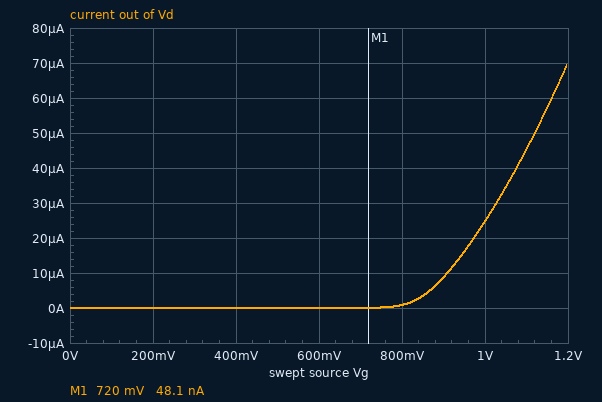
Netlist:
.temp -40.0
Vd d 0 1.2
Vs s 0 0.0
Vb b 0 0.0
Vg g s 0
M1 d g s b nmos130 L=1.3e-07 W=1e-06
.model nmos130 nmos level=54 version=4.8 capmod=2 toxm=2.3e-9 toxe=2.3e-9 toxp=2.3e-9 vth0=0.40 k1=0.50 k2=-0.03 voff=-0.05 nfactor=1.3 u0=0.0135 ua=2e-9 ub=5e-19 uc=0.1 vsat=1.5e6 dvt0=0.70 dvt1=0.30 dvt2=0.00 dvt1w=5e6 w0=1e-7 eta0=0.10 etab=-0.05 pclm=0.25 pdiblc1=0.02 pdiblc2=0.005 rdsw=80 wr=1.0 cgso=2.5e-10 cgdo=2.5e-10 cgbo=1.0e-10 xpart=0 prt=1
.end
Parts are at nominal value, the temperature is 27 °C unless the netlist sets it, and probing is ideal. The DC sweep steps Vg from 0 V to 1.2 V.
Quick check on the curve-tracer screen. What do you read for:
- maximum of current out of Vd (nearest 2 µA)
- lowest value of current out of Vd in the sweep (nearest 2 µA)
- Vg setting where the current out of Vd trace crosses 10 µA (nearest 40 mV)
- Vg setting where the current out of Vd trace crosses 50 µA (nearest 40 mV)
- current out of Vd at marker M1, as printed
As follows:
70 µA
0 A
920 mV
1.12 V
48.1 nA
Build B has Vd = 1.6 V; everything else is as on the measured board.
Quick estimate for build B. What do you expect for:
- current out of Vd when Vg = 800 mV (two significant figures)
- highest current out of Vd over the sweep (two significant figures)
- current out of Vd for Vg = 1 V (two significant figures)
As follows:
1.0 µA
72 µA
26 µA
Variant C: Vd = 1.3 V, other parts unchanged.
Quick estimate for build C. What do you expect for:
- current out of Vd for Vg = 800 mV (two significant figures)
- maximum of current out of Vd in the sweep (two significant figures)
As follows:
900 nA
71 µA
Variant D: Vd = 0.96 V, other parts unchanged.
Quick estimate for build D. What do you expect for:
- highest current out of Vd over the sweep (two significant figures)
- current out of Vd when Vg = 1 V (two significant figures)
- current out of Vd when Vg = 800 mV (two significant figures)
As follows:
69 µA
24 µA
800 nA
